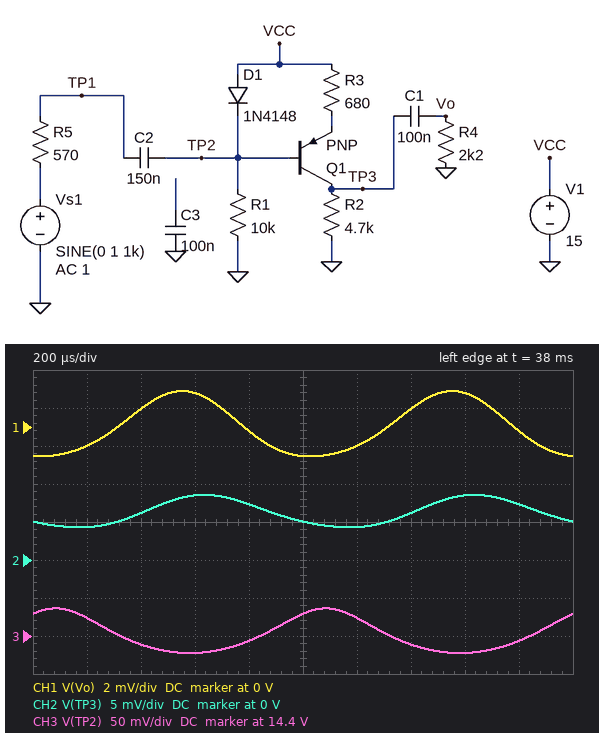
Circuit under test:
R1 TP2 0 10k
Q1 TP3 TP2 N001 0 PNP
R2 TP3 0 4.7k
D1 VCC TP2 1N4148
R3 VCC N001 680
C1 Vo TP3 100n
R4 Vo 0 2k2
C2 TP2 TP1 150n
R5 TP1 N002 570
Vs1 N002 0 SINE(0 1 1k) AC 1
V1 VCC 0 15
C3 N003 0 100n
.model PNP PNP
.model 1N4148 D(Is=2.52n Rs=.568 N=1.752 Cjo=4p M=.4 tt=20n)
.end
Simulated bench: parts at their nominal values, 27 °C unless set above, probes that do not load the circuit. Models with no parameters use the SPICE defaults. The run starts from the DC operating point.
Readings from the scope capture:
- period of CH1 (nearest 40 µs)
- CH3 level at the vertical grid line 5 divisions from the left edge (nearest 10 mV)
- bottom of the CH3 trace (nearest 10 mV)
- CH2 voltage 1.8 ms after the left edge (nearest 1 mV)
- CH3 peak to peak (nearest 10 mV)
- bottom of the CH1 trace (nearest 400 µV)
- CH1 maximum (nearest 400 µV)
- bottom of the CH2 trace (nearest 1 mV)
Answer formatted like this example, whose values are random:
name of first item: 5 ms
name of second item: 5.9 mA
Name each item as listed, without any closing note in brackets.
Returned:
period of CH1: 1.00 ms
CH3 level at the vertical grid line 5 divisions from the left edge: 14.43 V
bottom of the CH3 trace: 14.38 V
CH2 voltage 1.8 ms after the left edge: 7 mV
CH3 peak to peak: 60 mV
bottom of the CH1 trace: -1.6 mV
CH1 maximum: 2.0 mV
bottom of the CH2 trace: 4 mV
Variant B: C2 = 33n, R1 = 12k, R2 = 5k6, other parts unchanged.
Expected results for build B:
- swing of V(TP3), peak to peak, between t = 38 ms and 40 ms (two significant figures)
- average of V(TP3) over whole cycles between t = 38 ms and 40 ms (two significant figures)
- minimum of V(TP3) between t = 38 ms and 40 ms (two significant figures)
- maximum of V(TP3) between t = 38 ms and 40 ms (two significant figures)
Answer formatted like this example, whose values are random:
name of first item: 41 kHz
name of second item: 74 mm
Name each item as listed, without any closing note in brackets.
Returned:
swing of V(TP3), peak to peak, between t = 38 ms and 40 ms: 1.0 mV
average of V(TP3) over whole cycles between t = 38 ms and 40 ms: 5.0 mV
minimum of V(TP3) between t = 38 ms and 40 ms: 4.5 mV
maximum of V(TP3) between t = 38 ms and 40 ms: 5.5 mV
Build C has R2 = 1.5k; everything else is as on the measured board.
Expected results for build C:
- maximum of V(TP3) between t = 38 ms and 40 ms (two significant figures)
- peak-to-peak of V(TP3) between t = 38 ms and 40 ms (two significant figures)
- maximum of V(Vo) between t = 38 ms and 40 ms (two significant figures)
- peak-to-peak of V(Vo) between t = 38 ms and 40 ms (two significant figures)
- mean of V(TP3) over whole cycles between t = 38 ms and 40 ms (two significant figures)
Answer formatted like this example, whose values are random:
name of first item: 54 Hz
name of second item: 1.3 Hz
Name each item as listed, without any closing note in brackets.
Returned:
maximum of V(TP3) between t = 38 ms and 40 ms: 3.3 mV
peak-to-peak of V(TP3) between t = 38 ms and 40 ms: 2.4 mV
maximum of V(Vo) between t = 38 ms and 40 ms: 1.1 mV
peak-to-peak of V(Vo) between t = 38 ms and 40 ms: 1.9 mV
mean of V(TP3) over whole cycles between t = 38 ms and 40 ms: 2.0 mV
